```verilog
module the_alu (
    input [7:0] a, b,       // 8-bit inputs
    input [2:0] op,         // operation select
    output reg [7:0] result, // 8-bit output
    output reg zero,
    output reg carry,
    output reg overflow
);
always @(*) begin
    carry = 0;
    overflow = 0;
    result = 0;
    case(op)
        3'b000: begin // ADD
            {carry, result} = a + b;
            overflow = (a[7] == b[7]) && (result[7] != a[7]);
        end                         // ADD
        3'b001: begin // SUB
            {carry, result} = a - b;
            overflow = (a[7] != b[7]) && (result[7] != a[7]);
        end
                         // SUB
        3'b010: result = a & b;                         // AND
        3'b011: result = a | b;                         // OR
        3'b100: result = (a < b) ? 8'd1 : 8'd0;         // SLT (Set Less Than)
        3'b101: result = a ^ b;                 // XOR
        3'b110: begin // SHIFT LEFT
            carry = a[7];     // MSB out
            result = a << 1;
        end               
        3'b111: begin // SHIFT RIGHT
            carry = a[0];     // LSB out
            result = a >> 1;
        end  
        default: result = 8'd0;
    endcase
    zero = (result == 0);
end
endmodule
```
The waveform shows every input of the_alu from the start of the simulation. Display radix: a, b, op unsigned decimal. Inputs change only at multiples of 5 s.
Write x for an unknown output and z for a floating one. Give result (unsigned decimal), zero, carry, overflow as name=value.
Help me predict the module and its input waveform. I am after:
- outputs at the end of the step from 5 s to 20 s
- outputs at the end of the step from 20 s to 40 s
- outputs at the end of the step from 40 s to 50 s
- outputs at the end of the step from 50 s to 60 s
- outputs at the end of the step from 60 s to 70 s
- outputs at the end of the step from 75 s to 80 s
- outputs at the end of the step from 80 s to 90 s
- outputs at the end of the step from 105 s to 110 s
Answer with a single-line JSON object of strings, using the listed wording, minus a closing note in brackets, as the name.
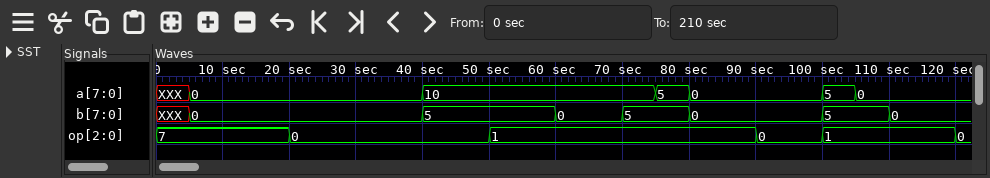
{"outputs at the end of the step from 5 s to 20 s": "result=0, zero=1, carry=0, overflow=0", "outputs at the end of the step from 20 s to 40 s": "result=0, zero=1, carry=0, overflow=0", "outputs at the end of the step from 40 s to 50 s": "result=15, zero=0, carry=0, overflow=0", "outputs at the end of the step from 50 s to 60 s": "result=5, zero=0, carry=0, overflow=0", "outputs at the end of the step from 60 s to 70 s": "result=10, zero=0, carry=0, overflow=0", "outputs at the end of the step from 75 s to 80 s": "result=0, zero=1, carry=0, overflow=0", "outputs at the end of the step from 80 s to 90 s": "result=0, zero=1, carry=0, overflow=0", "outputs at the end of the step from 105 s to 110 s": "result=251, zero=0, carry=1, overflow=0"}
